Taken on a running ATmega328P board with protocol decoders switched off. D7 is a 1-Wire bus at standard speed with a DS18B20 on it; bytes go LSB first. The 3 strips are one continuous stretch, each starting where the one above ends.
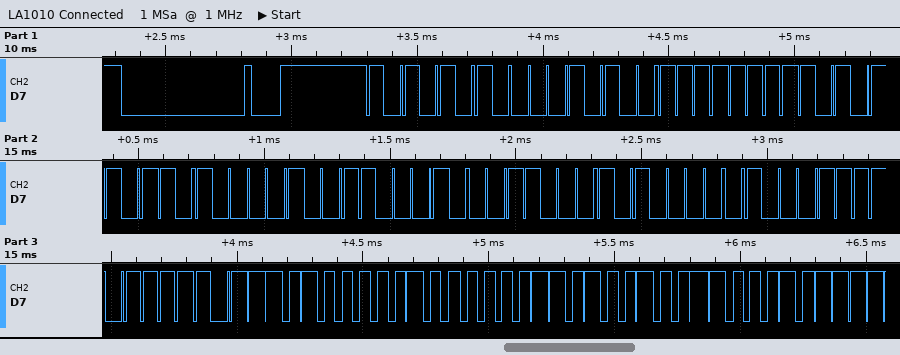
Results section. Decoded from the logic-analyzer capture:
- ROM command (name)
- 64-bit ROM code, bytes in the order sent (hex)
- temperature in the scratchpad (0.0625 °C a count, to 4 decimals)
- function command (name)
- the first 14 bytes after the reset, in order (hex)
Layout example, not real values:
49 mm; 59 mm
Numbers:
Match ROM; 28 FF B5 85 8C 18 05 F1; 32.6875 °C; Read Scratchpad; 55 28 FF B5 85 8C 18 05 F1 BE 0B 02 4B 46
